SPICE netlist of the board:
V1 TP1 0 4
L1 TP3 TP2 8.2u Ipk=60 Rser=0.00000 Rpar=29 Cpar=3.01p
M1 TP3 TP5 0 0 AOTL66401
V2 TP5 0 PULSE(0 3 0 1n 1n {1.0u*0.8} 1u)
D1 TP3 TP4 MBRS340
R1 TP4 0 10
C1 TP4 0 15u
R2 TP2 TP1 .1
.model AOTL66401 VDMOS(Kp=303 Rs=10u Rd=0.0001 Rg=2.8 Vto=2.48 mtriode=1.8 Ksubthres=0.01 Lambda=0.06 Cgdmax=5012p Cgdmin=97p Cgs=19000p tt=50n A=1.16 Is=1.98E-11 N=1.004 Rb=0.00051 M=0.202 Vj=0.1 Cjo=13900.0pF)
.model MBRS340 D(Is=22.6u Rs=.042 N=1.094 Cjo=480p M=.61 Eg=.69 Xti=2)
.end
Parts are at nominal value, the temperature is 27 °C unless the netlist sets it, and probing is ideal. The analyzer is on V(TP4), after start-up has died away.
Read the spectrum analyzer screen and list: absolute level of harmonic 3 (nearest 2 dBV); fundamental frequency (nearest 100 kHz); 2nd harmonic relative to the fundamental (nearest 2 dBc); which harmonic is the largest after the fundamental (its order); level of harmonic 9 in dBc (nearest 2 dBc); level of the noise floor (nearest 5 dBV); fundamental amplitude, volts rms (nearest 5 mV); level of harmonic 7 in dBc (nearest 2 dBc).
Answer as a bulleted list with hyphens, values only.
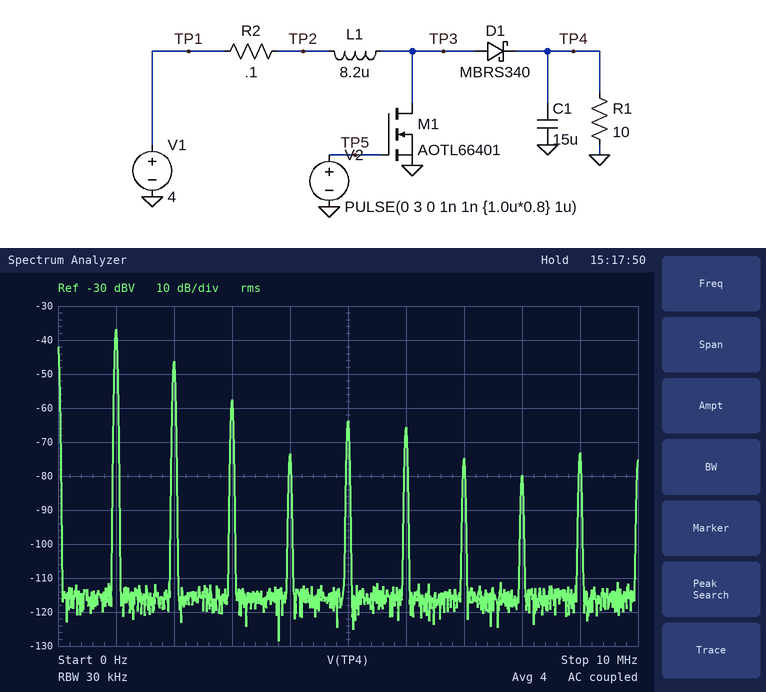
- -58 dBV
- 1.0 MHz
- -10 dBc
- 2
- -36 dBc
- -115 dBV
- 15 mV
- -38 dBc
